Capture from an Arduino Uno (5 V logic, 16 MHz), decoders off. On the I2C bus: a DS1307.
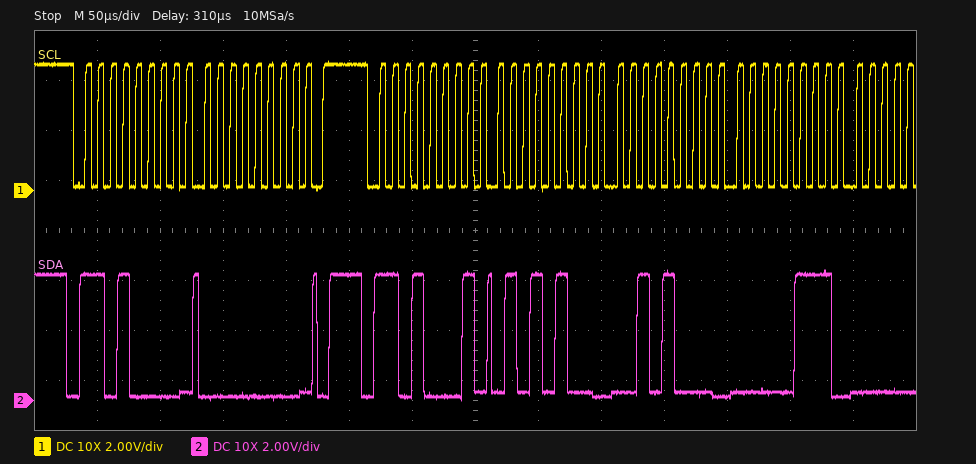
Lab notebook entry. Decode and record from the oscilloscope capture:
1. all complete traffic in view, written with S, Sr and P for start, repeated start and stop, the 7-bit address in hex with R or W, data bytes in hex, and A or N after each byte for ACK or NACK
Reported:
S 68W A 00 A P S 68R A 54 A 28 A 07 A
